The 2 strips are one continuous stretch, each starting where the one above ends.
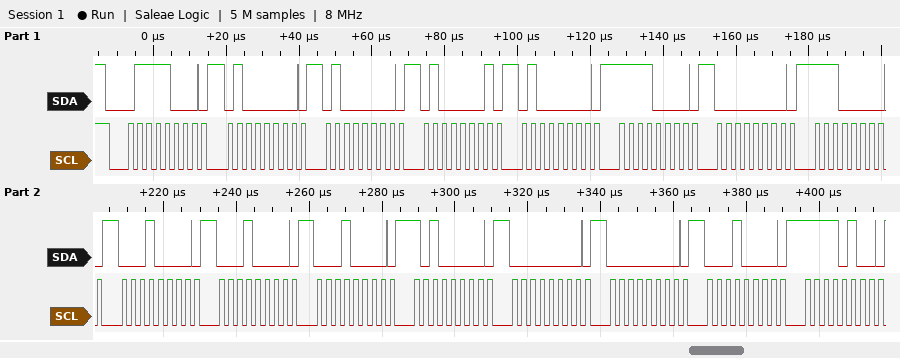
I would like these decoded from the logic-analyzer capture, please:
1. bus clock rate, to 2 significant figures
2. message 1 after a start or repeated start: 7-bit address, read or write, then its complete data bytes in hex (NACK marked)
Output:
400 kHz
0x3C write: 40 40 41 40 F0 00 E0 10 10 10 A0 00 00 10 F4
